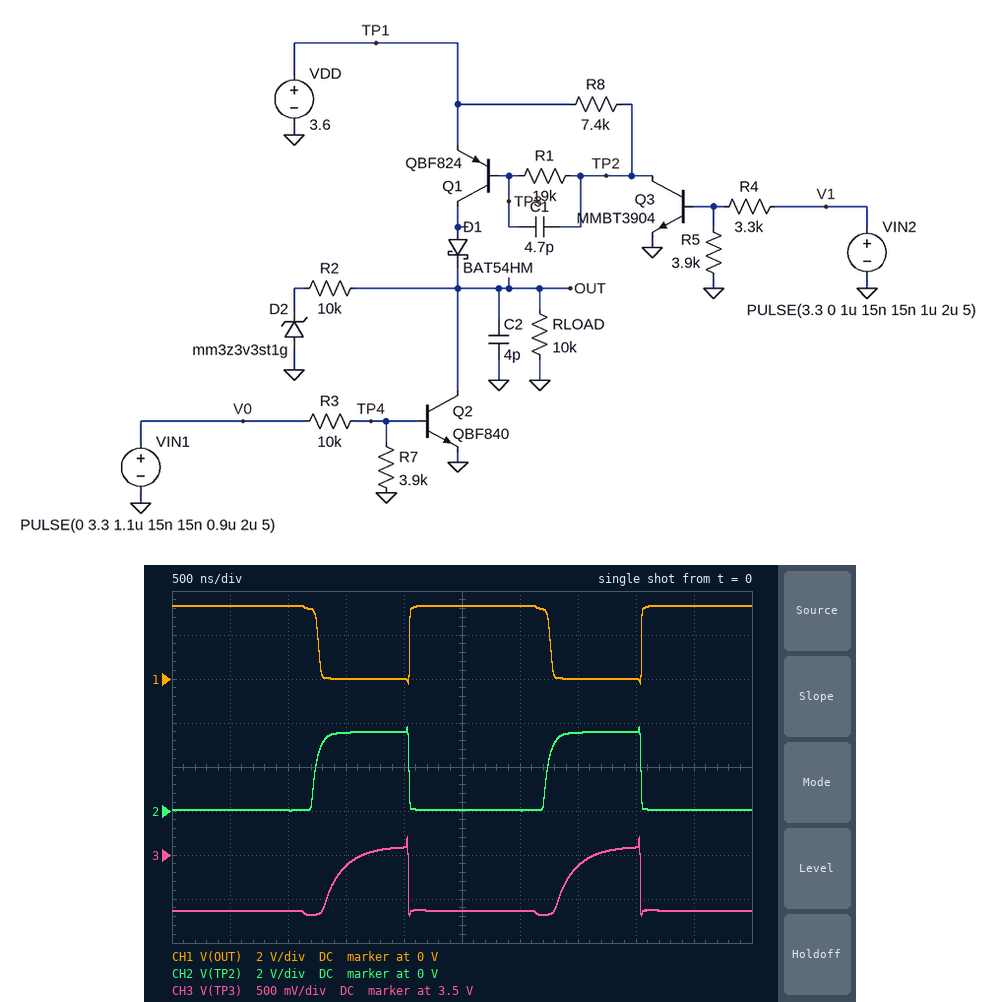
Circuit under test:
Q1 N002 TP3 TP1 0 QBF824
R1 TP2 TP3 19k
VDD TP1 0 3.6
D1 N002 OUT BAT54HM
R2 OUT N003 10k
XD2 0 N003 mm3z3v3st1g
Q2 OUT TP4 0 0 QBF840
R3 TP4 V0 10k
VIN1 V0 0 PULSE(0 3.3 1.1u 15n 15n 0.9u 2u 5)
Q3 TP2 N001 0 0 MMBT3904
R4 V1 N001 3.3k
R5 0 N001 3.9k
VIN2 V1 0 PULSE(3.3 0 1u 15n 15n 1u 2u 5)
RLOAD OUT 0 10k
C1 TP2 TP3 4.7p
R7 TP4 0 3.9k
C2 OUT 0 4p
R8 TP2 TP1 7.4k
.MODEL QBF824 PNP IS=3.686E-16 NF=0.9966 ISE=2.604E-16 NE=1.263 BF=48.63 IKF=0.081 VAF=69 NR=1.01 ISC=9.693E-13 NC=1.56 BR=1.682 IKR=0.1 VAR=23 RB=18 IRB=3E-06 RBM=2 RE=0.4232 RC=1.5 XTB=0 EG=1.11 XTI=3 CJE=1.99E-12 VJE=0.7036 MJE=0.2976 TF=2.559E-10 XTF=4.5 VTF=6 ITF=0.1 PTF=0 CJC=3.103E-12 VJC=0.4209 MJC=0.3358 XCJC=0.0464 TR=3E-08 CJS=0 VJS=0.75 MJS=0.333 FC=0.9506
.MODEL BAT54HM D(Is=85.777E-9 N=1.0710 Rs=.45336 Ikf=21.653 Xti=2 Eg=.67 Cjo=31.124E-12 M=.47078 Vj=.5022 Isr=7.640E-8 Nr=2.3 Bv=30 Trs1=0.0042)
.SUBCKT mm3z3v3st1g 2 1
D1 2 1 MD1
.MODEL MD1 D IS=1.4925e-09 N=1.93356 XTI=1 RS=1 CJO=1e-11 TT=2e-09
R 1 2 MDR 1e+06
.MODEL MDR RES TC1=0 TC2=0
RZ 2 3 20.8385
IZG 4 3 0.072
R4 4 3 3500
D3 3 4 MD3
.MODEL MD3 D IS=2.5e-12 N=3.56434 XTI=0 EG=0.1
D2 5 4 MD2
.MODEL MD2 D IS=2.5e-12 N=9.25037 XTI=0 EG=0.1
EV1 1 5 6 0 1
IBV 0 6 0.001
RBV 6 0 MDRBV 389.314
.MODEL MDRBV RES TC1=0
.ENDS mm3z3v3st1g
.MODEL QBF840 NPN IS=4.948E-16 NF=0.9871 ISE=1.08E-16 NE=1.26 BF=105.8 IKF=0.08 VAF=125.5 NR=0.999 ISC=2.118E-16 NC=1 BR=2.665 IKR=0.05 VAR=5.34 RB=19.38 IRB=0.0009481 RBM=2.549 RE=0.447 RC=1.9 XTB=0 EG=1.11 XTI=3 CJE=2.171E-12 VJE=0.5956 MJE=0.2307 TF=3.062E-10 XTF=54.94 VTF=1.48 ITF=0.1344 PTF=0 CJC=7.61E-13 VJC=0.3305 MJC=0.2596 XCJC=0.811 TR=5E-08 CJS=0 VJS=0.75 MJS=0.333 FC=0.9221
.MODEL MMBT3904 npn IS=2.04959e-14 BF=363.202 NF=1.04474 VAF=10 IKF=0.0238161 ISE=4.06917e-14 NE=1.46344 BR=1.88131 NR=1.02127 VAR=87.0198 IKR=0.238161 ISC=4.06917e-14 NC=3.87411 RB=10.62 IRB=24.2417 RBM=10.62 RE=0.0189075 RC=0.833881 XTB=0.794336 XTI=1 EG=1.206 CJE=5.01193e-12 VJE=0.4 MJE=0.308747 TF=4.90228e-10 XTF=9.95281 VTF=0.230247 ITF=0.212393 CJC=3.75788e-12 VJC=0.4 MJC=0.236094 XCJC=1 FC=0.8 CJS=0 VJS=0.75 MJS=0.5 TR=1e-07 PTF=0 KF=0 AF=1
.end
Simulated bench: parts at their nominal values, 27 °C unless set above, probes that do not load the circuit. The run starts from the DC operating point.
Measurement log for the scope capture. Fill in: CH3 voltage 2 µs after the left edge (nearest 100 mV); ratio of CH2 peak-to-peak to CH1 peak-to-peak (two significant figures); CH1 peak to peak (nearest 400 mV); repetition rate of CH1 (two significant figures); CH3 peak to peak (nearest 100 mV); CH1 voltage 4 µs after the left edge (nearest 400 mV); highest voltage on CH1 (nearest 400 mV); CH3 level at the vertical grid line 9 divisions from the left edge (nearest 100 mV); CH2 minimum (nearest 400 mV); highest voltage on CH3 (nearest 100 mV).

3.6 V
1.1
3.6 V
500 kHz
900 mV
0 V
3.2 V
2.9 V
0 V
3.7 V
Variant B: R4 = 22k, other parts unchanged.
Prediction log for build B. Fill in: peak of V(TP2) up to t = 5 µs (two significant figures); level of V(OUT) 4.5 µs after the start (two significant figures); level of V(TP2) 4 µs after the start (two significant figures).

3.7 V
-18 mV
3.6 V
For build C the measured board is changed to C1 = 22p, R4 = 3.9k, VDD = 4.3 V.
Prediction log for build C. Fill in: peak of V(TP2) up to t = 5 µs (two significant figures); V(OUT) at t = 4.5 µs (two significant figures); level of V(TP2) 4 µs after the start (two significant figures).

4.5 V
4.0 V
4.3 V
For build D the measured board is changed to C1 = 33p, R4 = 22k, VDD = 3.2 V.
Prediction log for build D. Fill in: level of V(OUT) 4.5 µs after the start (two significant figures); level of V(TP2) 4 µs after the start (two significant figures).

-18 mV
3.2 V
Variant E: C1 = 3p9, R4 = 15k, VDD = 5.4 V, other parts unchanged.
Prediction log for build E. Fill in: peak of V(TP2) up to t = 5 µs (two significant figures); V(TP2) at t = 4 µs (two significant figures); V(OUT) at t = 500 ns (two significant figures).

5.5 V
5.4 V
5.1 V
